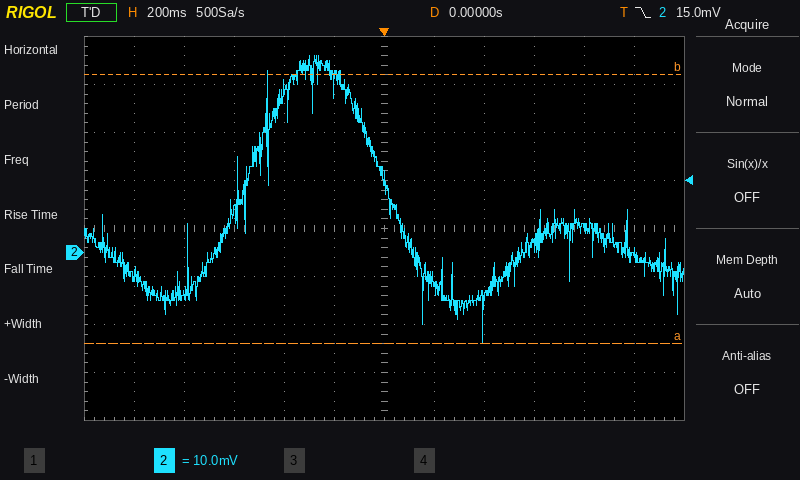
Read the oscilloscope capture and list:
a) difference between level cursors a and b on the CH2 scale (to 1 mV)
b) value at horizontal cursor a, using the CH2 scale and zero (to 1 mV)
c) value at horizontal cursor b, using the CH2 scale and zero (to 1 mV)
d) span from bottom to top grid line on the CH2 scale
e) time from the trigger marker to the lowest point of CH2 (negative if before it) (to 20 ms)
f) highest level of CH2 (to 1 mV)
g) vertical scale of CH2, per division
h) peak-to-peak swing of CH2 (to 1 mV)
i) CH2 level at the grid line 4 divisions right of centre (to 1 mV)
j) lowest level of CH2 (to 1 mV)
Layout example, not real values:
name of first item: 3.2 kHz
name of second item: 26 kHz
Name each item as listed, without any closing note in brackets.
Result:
difference between level cursors a and b on the CH2 scale: 56 mV
value at horizontal cursor a, using the CH2 scale and zero: -19 mV
value at horizontal cursor b, using the CH2 scale and zero: 37 mV
span from bottom to top grid line on the CH2 scale: 80 mV
time from the trigger marker to the lowest point of CH2 (negative if before it): +400 ms
highest level of CH2: 41 mV
vertical scale of CH2, per division: 10 mV
peak-to-peak swing of CH2: 60 mV
CH2 level at the grid line 4 divisions right of centre: 5 mV
lowest level of CH2: -19 mV
